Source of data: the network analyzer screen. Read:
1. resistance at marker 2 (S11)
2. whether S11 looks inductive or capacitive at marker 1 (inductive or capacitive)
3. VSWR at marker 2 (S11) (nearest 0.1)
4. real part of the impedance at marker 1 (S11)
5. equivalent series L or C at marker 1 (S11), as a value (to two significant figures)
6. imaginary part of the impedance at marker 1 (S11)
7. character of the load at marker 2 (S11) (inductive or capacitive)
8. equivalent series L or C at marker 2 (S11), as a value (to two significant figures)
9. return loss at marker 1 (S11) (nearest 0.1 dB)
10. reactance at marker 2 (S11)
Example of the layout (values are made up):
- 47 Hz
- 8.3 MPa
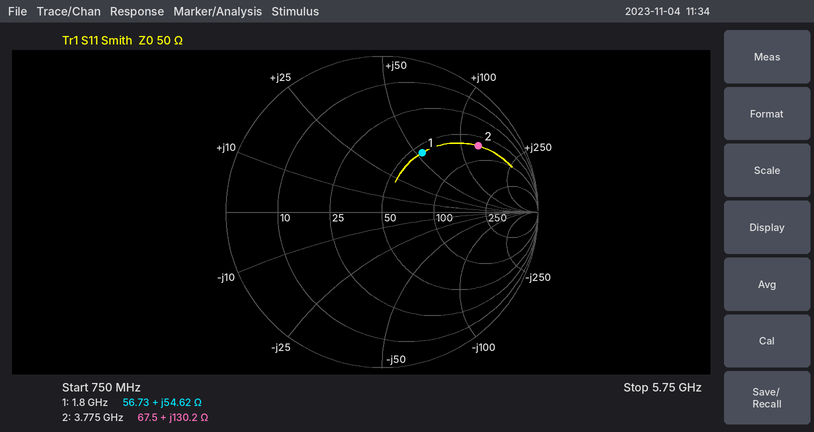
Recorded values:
- 67.5 Ω
- inductive
- 7.0
- 56.73 Ω
- 4.8 nH
- +54.62 Ω
- inductive
- 5.5 nH
- 6.8 dB
- +130.2 Ω
